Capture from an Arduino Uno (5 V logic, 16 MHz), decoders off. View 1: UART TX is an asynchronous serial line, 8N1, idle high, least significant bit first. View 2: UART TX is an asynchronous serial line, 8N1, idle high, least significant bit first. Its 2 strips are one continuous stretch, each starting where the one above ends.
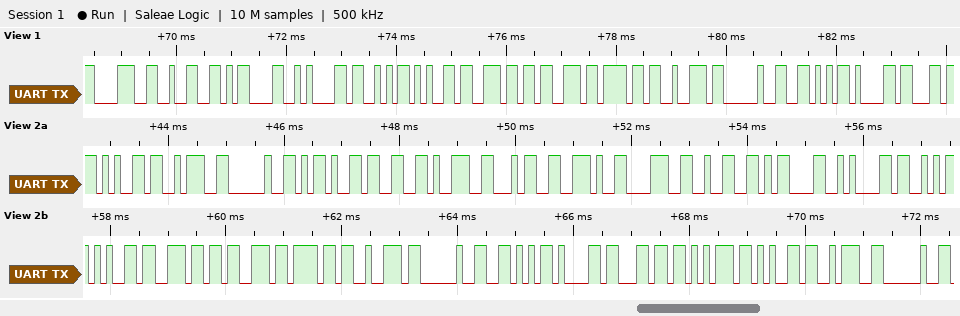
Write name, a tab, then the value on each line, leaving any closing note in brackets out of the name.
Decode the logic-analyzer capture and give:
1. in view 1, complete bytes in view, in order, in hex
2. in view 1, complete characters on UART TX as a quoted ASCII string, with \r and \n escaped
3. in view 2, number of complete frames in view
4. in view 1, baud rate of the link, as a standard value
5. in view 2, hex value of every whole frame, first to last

in view 1, complete bytes in view, in order, in hex	0x38 0x32 0x0D 0x0A 0x53 0x65 0x6E 0x73 0x6F 0x72 0x20 0x56 0x61
in view 1, complete characters on UART TX as a quoted ASCII string, with \r and \n escaped	"82\r\nSensor Va"
in view 2, number of complete frames in view	26
in view 1, baud rate of the link, as a standard value	9600 baud
in view 2, hex value of every whole frame, first to last	0x65 0x3A 0x20 0x2D 0x33 0x39 0x34 0x2E 0x38 0x32 0x0D 0x0A 0x53 0x65 0x6E 0x73 0x6F 0x72 0x20 0x56 0x61 0x6C 0x75 0x65 0x3A 0x20
